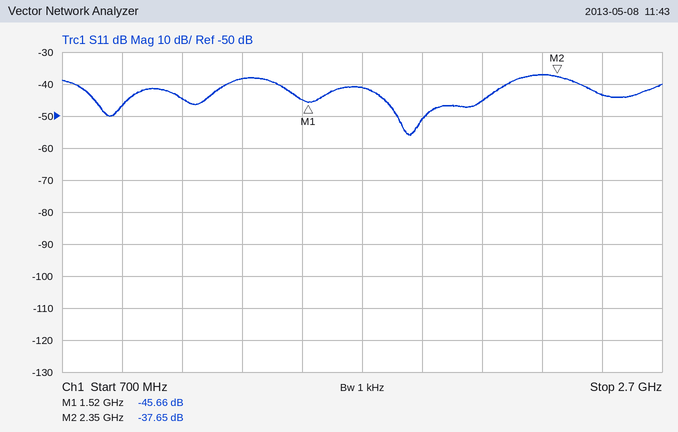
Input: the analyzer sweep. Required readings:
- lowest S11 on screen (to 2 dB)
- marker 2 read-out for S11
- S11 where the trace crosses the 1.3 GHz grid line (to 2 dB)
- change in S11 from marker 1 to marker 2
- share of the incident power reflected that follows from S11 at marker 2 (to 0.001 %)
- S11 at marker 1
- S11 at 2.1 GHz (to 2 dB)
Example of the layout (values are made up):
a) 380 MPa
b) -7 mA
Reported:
a) -56 dB
b) -37.65 dB
c) -38 dB
d) 8.01 dB
e) 0.017 %
f) -45.66 dB
g) -46 dB
